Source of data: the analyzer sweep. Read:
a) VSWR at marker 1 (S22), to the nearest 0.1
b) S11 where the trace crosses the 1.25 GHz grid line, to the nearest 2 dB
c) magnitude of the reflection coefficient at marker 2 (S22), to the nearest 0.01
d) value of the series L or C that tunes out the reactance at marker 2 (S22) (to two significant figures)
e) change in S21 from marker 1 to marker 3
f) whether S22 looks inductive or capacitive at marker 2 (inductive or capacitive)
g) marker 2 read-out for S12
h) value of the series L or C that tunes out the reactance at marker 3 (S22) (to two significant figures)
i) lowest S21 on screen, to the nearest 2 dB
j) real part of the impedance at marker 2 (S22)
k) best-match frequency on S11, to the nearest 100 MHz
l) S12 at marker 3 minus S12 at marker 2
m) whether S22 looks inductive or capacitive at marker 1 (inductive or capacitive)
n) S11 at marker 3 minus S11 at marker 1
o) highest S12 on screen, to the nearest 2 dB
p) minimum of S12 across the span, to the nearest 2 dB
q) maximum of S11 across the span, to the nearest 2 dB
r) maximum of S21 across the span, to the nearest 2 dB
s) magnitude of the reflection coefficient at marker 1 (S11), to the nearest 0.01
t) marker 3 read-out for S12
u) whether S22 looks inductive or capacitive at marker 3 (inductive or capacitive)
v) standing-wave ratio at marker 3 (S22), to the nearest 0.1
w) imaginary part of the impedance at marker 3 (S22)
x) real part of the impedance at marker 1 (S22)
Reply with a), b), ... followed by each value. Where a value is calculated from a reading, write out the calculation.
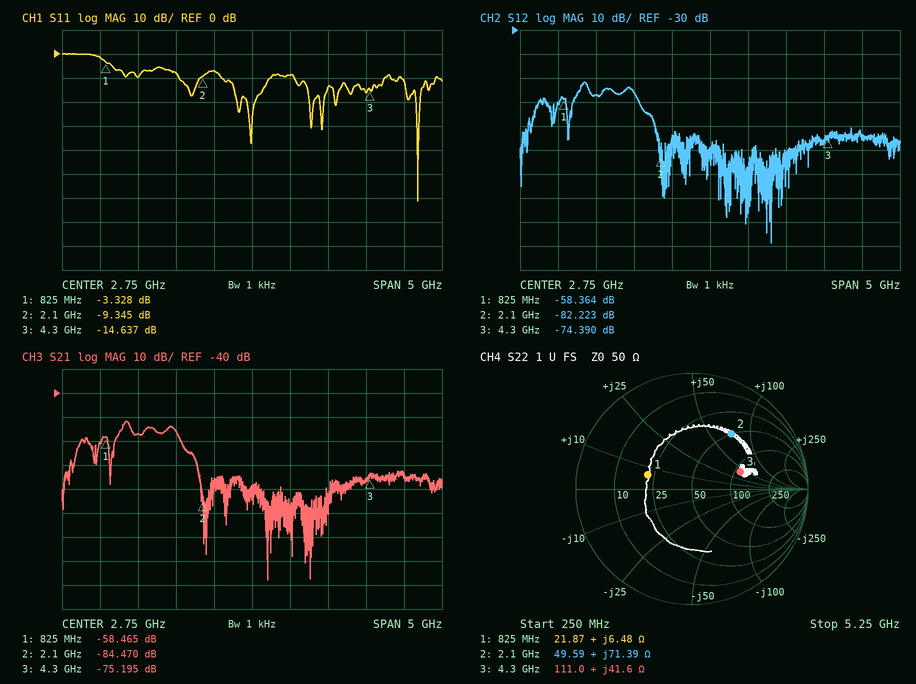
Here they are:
a) 2.3
b) -10 dB
c) 0.58
d) C = 1/(2π × 2.1 GHz × 71.39 Ω) ≈ 1.1 pF
e) -75.195 − (-58.465) = -16.730 dB
f) inductive
g) -82.223 dB
h) C = 1/(2π × 4.3 GHz × 41.6 Ω) ≈ 890 fF
i) -118 dB
j) 49.59 Ω
k) 4.9 GHz
l) -74.39 − (-82.223) = 7.833 dB
m) inductive
n) -14.637 − (-3.328) = -11.309 dB
o) -52 dB
p) -118 dB
q) 0 dB
r) -52 dB
s) 10^(-3.328/20) ≈ 0.68
t) -74.390 dB
u) inductive
v) 2.6
w) +41.6 Ω
x) 21.87 Ω
